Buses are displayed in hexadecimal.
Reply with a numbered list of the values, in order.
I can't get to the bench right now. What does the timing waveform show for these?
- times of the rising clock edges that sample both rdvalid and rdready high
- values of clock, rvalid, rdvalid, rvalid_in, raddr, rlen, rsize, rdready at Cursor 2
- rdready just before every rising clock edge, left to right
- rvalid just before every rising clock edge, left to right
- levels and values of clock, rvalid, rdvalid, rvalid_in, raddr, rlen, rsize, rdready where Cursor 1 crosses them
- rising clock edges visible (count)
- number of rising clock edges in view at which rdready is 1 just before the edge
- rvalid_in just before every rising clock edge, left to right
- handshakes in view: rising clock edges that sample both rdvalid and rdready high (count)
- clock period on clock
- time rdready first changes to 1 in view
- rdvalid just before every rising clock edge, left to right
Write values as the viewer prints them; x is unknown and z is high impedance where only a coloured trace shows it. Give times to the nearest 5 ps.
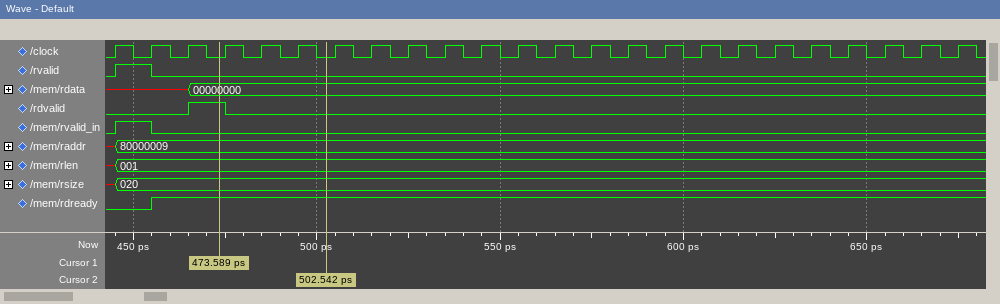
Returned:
1. 475 ps
2. clock=0, rvalid=0, rdvalid=0, rvalid_in=0, raddr=80000009, rlen=001, rsize=020, rdready=1
3. 0 0 1 1 1 1 1 1 1 1 1 1 1 1 1 1 1 1 1 1 1 1 1 1
4. 0 1 0 0 0 0 0 0 0 0 0 0 0 0 0 0 0 0 0 0 0 0 0 0
5. clock=0, rvalid=0, rdvalid=1, rvalid_in=0, raddr=80000009, rlen=001, rsize=020, rdready=1
6. 24
7. 22
8. 0 1 0 0 0 0 0 0 0 0 0 0 0 0 0 0 0 0 0 0 0 0 0 0
9. 1
10. 10 ps
11. 455 ps
12. 0 0 0 1 0 0 0 0 0 0 0 0 0 0 0 0 0 0 0 0 0 0 0 0
